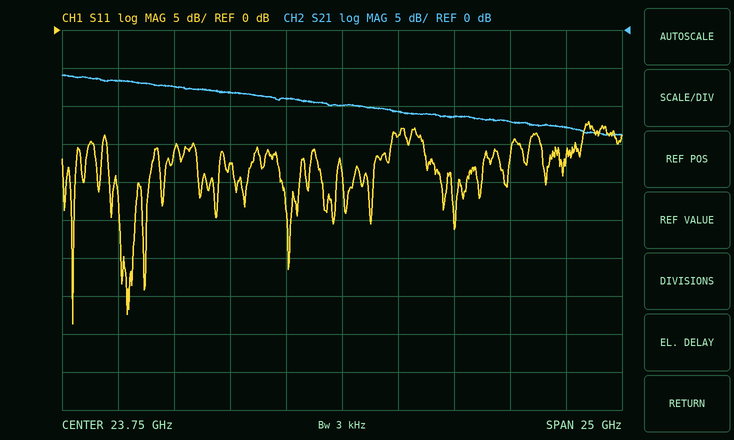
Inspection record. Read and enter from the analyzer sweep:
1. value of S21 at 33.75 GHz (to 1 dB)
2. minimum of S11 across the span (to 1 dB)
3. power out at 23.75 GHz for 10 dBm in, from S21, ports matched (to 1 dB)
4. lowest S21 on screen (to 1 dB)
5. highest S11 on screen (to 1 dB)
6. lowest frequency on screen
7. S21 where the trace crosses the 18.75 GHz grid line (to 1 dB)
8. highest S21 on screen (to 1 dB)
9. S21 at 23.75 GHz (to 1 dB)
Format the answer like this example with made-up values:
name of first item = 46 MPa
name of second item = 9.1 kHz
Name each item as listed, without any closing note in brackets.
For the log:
value of S21 at 33.75 GHz = -13 dB
minimum of S11 across the span = -39 dB
power out at 23.75 GHz for 10 dBm in, from S21, ports matched = 0 dBm
lowest S21 on screen = -14 dB
highest S11 on screen = -12 dB
lowest frequency on screen = 11.25 GHz
S21 where the trace crosses the 18.75 GHz grid line = -8 dB
highest S21 on screen = -6 dB
S21 at 23.75 GHz = -10 dB
